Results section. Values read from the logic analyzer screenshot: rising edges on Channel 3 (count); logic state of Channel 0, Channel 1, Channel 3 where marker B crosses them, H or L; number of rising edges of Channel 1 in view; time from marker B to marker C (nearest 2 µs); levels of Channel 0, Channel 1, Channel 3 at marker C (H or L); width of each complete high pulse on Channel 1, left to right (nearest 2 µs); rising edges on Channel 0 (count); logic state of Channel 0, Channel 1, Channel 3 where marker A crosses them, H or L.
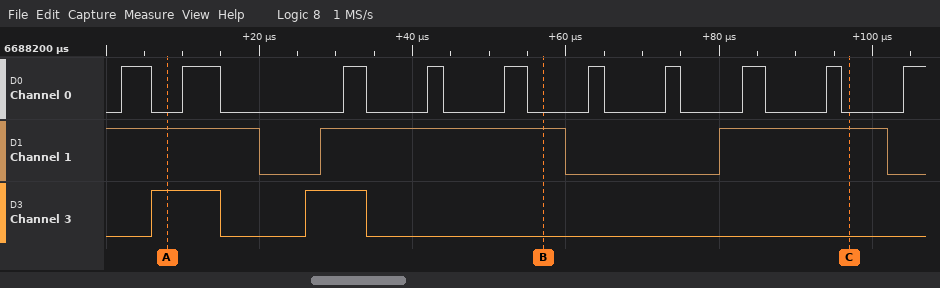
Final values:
2
Channel 0=L, Channel 1=H, Channel 3=L
2
40 µs
Channel 0=L, Channel 1=H, Channel 3=L
32 µs, 22 µs
10
Channel 0=L, Channel 1=H, Channel 3=H
